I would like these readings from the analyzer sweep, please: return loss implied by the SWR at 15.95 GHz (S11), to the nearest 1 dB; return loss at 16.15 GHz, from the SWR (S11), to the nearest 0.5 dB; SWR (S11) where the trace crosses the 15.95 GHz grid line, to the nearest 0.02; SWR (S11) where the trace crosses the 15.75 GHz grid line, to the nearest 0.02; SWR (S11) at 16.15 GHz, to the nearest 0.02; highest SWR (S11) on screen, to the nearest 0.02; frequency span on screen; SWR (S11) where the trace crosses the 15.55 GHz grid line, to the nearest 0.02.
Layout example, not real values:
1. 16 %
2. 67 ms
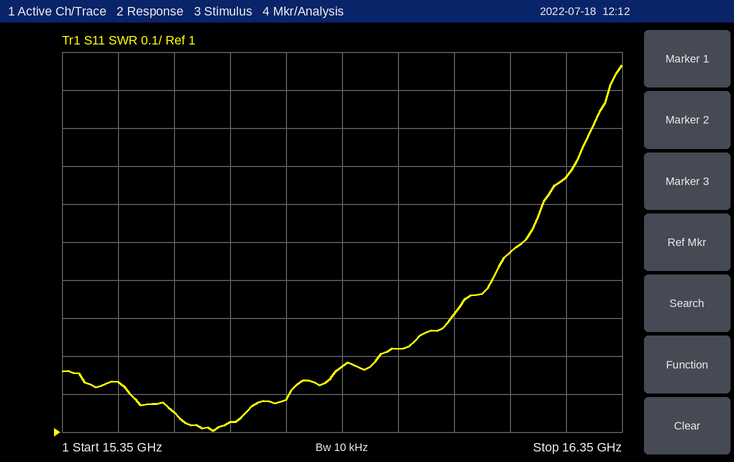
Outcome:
1. 20 dB
2. 14.5 dB
3. 1.22
4. 1.08
5. 1.48
6. 1.96
7. 1 GHz
8. 1.06
